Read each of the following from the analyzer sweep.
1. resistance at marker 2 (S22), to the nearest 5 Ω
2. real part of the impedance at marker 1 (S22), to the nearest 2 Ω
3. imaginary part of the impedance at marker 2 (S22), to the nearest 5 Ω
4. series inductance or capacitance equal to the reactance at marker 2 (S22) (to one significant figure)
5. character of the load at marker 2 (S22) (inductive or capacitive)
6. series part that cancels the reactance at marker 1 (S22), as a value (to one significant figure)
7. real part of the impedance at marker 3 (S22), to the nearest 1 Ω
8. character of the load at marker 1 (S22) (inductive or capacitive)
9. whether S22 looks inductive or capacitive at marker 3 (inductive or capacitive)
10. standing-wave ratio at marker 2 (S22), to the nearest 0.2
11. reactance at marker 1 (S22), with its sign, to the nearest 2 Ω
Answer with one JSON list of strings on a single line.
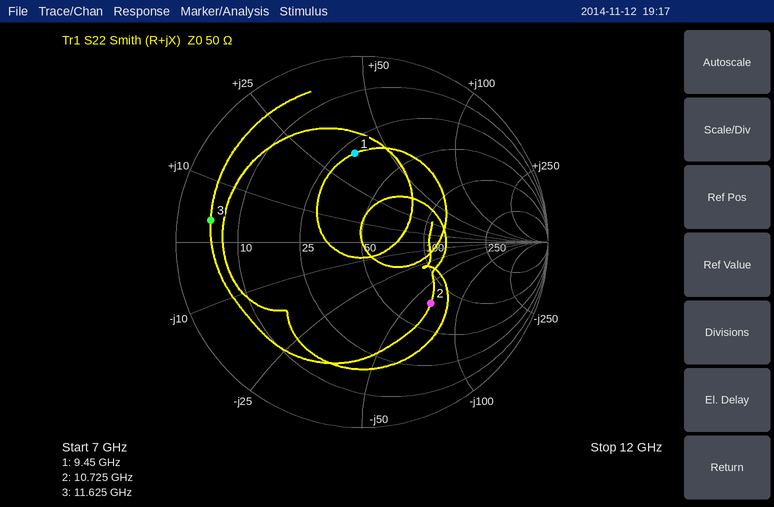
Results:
["75 Ω", "30 Ω", "-65 Ω", "200 fF", "capacitive", "500 fF", "5 Ω", "inductive", "inductive", "3.0", "+36 Ω"]
